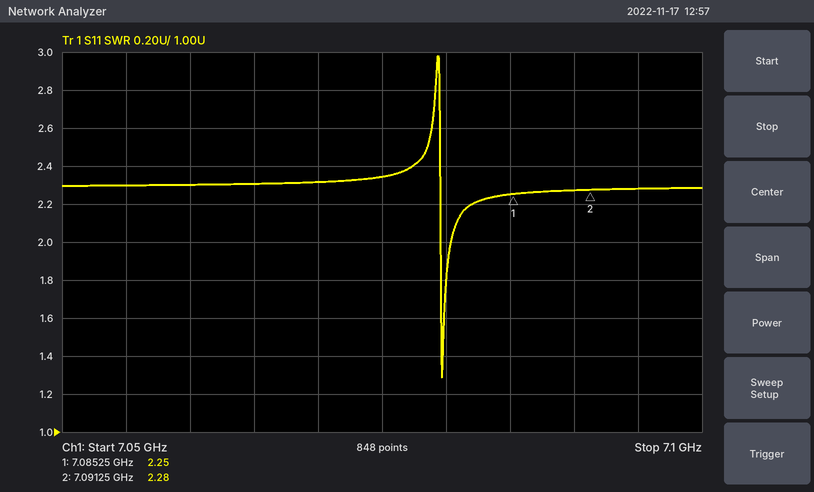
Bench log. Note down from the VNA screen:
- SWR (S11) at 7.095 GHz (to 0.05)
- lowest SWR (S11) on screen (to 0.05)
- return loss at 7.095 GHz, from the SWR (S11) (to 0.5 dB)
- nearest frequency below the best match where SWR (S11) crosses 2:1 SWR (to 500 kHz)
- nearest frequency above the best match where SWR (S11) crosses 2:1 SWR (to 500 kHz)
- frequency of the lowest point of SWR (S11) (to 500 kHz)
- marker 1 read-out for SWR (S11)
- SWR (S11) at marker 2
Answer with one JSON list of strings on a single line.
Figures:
["2.30", "1.30", "8.0 dB", "7.0795 GHz", "7.0805 GHz", "7.0795 GHz", "2.25", "2.28"]
